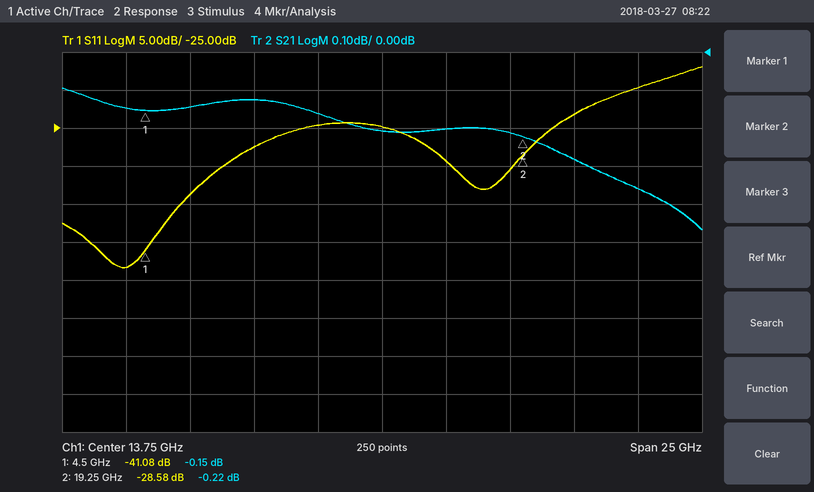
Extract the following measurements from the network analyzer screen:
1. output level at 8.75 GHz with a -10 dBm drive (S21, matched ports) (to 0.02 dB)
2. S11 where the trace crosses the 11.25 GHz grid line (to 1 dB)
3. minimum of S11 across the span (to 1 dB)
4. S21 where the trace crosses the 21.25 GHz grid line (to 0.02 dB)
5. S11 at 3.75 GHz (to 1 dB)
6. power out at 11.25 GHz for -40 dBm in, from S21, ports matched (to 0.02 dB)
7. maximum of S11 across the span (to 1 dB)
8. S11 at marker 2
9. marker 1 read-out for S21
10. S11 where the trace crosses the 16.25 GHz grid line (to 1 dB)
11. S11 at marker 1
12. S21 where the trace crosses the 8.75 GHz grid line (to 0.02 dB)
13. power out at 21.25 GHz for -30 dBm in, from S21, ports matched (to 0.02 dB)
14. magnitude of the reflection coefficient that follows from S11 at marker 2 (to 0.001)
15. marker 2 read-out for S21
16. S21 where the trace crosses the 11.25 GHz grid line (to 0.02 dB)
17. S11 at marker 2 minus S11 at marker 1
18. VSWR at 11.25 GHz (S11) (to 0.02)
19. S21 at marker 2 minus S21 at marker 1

-10.12 dBm
-25 dB
-43 dB
-0.28 dB
-43 dB
-40.16 dBm
-17 dB
-28.58 dB
-0.15 dB
-29 dB
-41.08 dB
-0.12 dB
-30.28 dBm
0.037
-0.22 dB
-0.16 dB
12.50 dB
1.12
-0.07 dB
